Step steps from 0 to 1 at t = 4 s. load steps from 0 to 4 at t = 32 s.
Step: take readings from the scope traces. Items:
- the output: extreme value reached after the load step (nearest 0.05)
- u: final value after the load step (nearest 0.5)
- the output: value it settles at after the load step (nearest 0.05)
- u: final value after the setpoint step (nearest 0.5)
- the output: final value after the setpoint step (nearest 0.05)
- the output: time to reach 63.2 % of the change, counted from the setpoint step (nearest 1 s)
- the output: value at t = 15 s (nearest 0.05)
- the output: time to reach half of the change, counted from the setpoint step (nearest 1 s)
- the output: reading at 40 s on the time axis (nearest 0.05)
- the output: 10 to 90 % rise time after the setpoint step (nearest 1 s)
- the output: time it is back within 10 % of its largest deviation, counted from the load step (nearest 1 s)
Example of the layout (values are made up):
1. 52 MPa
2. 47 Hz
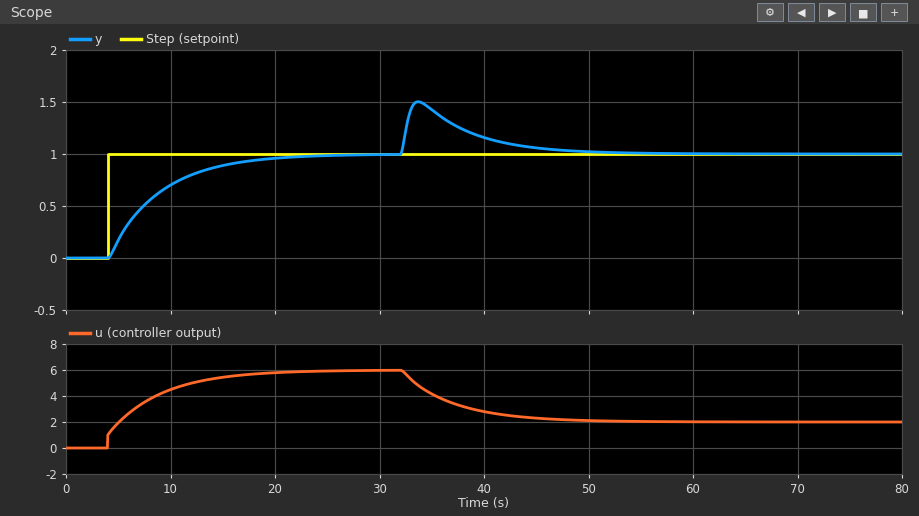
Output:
1. 1.50
2. 2.0
3. 1.00
4. 6.0
5. 1.00
6. 5 s
7. 0.90
8. 3 s
9. 1.15
10. 11 s
11. 14 s
